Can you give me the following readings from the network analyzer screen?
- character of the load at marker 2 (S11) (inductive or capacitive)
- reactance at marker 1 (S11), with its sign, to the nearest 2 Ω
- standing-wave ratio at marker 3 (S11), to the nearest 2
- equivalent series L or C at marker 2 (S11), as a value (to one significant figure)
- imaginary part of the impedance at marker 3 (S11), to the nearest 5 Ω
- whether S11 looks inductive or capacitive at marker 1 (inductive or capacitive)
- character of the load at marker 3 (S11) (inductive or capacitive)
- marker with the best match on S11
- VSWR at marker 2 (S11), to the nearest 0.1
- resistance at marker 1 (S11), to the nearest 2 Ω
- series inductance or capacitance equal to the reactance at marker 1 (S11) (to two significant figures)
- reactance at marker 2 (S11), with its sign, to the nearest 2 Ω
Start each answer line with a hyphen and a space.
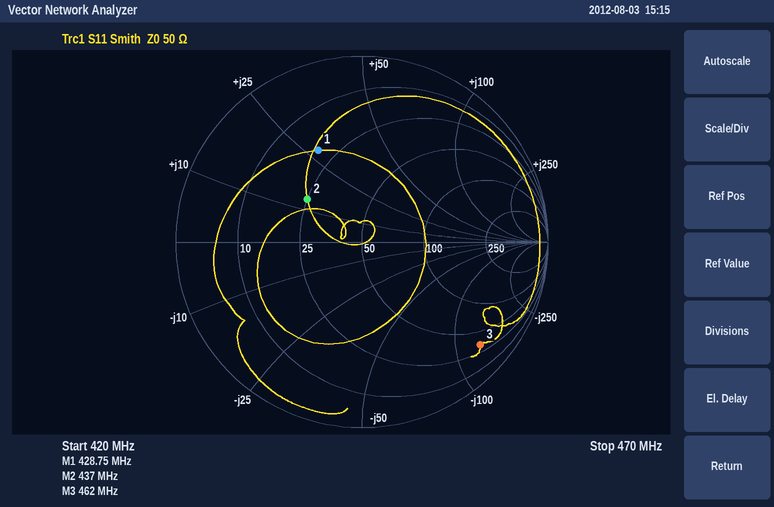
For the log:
- inductive
- +28 Ω
- 12
- 5 nH
- -125 Ω
- inductive
- capacitive
- marker 2
- 2.2
- 20 Ω
- 10 nH
- +14 Ω
